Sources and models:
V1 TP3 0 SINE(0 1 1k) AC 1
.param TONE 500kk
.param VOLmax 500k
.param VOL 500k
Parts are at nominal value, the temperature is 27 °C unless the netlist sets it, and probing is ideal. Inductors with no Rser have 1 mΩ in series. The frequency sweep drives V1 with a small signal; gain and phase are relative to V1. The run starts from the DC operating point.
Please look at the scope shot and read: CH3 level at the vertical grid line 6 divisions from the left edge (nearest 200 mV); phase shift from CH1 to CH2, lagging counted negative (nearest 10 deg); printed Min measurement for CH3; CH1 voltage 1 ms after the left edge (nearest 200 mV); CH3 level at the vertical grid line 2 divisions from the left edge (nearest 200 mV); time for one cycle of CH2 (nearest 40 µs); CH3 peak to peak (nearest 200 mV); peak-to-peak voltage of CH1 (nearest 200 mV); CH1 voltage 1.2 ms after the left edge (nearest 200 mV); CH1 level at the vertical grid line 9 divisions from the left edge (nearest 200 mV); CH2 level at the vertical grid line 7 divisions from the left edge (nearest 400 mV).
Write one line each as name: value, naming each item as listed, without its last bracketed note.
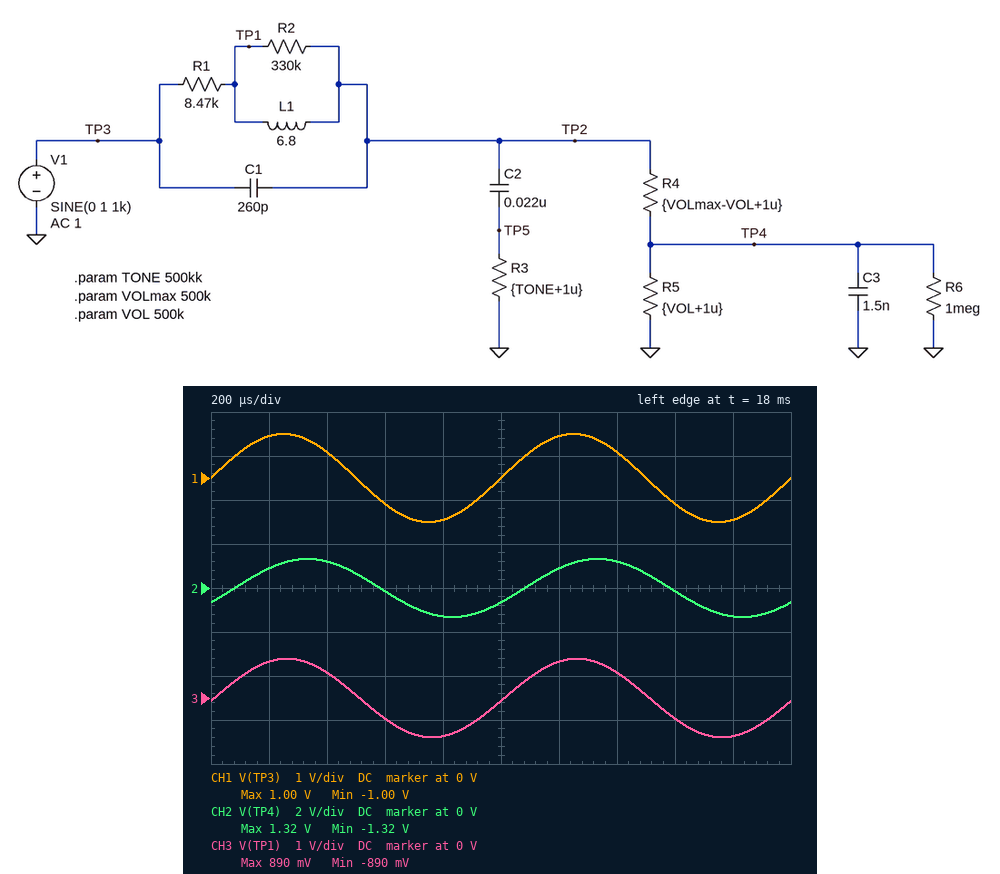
CH3 level at the vertical grid line 6 divisions from the left edge: 800 mV
phase shift from CH1 to CH2, lagging counted negative: -30 deg
printed Min measurement for CH3: -890 mV
CH1 voltage 1 ms after the left edge: 0 V
CH3 level at the vertical grid line 2 divisions from the left edge: 600 mV
time for one cycle of CH2: 1.00 ms
CH3 peak to peak: 1.8 V
peak-to-peak voltage of CH1: 2.0 V
CH1 voltage 1.2 ms after the left edge: 1.0 V
CH1 level at the vertical grid line 9 divisions from the left edge: -1.0 V
CH2 level at the vertical grid line 7 divisions from the left edge: 1.2 V
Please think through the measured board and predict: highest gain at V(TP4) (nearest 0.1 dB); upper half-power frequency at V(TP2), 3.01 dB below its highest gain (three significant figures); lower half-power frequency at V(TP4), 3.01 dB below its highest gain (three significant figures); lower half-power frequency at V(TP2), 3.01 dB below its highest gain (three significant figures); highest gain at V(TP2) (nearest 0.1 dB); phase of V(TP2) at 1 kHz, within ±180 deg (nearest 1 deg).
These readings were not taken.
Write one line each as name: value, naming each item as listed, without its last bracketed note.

highest gain at V(TP4): 3.3 dB
upper half-power frequency at V(TP2), 3.01 dB below its highest gain: 1.68 kHz
lower half-power frequency at V(TP4), 3.01 dB below its highest gain: 473 Hz
lower half-power frequency at V(TP2), 3.01 dB below its highest gain: 473 Hz
highest gain at V(TP2): 3.3 dB
phase of V(TP2) at 1 kHz, within ±180 deg: -30 deg
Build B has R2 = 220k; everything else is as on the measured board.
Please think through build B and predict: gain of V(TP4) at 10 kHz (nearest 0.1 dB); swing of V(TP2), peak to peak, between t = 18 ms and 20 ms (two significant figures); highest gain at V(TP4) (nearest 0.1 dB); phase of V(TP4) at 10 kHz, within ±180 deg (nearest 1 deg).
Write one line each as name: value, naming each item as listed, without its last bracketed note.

gain of V(TP4) at 10 kHz: -17.3 dB
swing of V(TP2), peak to peak, between t = 18 ms and 20 ms: 2.5 V
highest gain at V(TP4): 2.5 dB
phase of V(TP4) at 10 kHz, within ±180 deg: -12 deg
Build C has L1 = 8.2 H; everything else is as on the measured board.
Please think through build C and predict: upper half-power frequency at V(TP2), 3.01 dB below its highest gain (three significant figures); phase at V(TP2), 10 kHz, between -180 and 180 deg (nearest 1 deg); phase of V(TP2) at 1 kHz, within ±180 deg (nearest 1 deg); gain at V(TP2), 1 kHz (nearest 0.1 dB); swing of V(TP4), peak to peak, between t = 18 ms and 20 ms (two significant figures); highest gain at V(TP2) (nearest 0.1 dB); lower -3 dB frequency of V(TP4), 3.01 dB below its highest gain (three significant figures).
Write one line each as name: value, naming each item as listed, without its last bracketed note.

upper half-power frequency at V(TP2), 3.01 dB below its highest gain: 1.53 kHz
phase at V(TP2), 10 kHz, between -180 and 180 deg: -7 deg
phase of V(TP2) at 1 kHz, within ±180 deg: -38 deg
gain at V(TP2), 1 kHz: 2.6 dB
swing of V(TP4), peak to peak, between t = 18 ms and 20 ms: 2.7 V
highest gain at V(TP2): 2.9 dB
lower -3 dB frequency of V(TP4), 3.01 dB below its highest gain: 276 Hz
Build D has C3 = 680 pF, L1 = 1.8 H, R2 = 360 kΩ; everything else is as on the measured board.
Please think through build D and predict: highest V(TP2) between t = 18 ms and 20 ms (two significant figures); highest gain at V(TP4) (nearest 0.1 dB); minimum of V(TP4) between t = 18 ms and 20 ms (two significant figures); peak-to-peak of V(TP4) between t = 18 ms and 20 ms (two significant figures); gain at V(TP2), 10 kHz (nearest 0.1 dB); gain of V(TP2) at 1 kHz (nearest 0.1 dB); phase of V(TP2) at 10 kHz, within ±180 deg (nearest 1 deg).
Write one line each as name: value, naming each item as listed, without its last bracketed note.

highest V(TP2) between t = 18 ms and 20 ms: 1.0 V
highest gain at V(TP4): 3.4 dB
minimum of V(TP4) between t = 18 ms and 20 ms: -1.0 V
peak-to-peak of V(TP4) between t = 18 ms and 20 ms: 2.0 V
gain at V(TP2), 10 kHz: -15.5 dB
gain of V(TP2) at 1 kHz: 0 dB
phase of V(TP2) at 10 kHz, within ±180 deg: -13 deg
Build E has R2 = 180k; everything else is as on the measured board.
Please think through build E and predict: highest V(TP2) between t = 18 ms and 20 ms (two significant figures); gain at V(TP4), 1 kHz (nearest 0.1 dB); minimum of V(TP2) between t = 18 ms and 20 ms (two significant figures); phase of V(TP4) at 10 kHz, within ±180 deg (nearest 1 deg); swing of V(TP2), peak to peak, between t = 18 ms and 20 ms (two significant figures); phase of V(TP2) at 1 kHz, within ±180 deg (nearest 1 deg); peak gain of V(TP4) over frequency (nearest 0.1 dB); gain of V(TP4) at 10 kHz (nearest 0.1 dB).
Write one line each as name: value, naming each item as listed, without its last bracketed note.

highest V(TP2) between t = 18 ms and 20 ms: 1.2 V
gain at V(TP4), 1 kHz: 1.8 dB
minimum of V(TP2) between t = 18 ms and 20 ms: -1.2 V
phase of V(TP4) at 10 kHz, within ±180 deg: -15 deg
swing of V(TP2), peak to peak, between t = 18 ms and 20 ms: 2.5 V
phase of V(TP2) at 1 kHz, within ±180 deg: -30 deg
peak gain of V(TP4) over frequency: 2.1 dB
gain of V(TP4) at 10 kHz: -17.1 dB
